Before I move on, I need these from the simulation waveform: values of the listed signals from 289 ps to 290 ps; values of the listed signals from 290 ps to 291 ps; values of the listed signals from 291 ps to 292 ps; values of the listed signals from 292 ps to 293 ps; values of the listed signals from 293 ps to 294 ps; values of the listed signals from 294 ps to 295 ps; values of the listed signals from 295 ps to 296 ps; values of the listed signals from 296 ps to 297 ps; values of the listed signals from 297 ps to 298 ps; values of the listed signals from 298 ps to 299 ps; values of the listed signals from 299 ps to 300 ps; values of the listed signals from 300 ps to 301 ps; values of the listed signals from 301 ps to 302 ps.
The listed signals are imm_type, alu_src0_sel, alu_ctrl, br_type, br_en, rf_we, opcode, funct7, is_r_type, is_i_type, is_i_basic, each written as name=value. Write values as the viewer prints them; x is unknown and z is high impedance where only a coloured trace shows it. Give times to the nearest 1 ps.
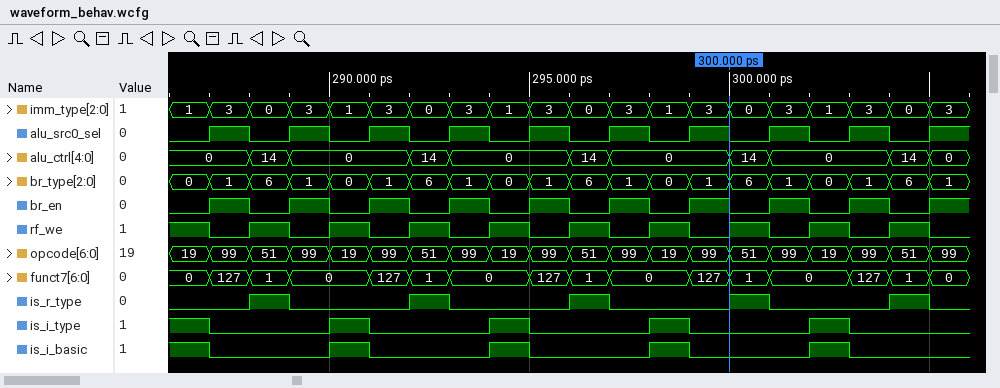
imm_type=3, alu_src0_sel=1, alu_ctrl=0, br_type=1, br_en=1, rf_we=0, opcode=99, funct7=0, is_r_type=0, is_i_type=0, is_i_basic=0
imm_type=1, alu_src0_sel=0, alu_ctrl=0, br_type=0, br_en=0, rf_we=1, opcode=19, funct7=0, is_r_type=0, is_i_type=1, is_i_basic=1
imm_type=3, alu_src0_sel=1, alu_ctrl=0, br_type=1, br_en=1, rf_we=0, opcode=99, funct7=127, is_r_type=0, is_i_type=0, is_i_basic=0
imm_type=0, alu_src0_sel=0, alu_ctrl=14, br_type=6, br_en=0, rf_we=1, opcode=51, funct7=1, is_r_type=1, is_i_type=0, is_i_basic=0
imm_type=3, alu_src0_sel=1, alu_ctrl=0, br_type=1, br_en=1, rf_we=0, opcode=99, funct7=0, is_r_type=0, is_i_type=0, is_i_basic=0
imm_type=1, alu_src0_sel=0, alu_ctrl=0, br_type=0, br_en=0, rf_we=1, opcode=19, funct7=0, is_r_type=0, is_i_type=1, is_i_basic=1
imm_type=3, alu_src0_sel=1, alu_ctrl=0, br_type=1, br_en=1, rf_we=0, opcode=99, funct7=127, is_r_type=0, is_i_type=0, is_i_basic=0
imm_type=0, alu_src0_sel=0, alu_ctrl=14, br_type=6, br_en=0, rf_we=1, opcode=51, funct7=1, is_r_type=1, is_i_type=0, is_i_basic=0
imm_type=3, alu_src0_sel=1, alu_ctrl=0, br_type=1, br_en=1, rf_we=0, opcode=99, funct7=0, is_r_type=0, is_i_type=0, is_i_basic=0
imm_type=1, alu_src0_sel=0, alu_ctrl=0, br_type=0, br_en=0, rf_we=1, opcode=19, funct7=0, is_r_type=0, is_i_type=1, is_i_basic=1
imm_type=3, alu_src0_sel=1, alu_ctrl=0, br_type=1, br_en=1, rf_we=0, opcode=99, funct7=127, is_r_type=0, is_i_type=0, is_i_basic=0
imm_type=0, alu_src0_sel=0, alu_ctrl=14, br_type=6, br_en=0, rf_we=1, opcode=51, funct7=1, is_r_type=1, is_i_type=0, is_i_basic=0
imm_type=3, alu_src0_sel=1, alu_ctrl=0, br_type=1, br_en=1, rf_we=0, opcode=99, funct7=0, is_r_type=0, is_i_type=0, is_i_basic=0
